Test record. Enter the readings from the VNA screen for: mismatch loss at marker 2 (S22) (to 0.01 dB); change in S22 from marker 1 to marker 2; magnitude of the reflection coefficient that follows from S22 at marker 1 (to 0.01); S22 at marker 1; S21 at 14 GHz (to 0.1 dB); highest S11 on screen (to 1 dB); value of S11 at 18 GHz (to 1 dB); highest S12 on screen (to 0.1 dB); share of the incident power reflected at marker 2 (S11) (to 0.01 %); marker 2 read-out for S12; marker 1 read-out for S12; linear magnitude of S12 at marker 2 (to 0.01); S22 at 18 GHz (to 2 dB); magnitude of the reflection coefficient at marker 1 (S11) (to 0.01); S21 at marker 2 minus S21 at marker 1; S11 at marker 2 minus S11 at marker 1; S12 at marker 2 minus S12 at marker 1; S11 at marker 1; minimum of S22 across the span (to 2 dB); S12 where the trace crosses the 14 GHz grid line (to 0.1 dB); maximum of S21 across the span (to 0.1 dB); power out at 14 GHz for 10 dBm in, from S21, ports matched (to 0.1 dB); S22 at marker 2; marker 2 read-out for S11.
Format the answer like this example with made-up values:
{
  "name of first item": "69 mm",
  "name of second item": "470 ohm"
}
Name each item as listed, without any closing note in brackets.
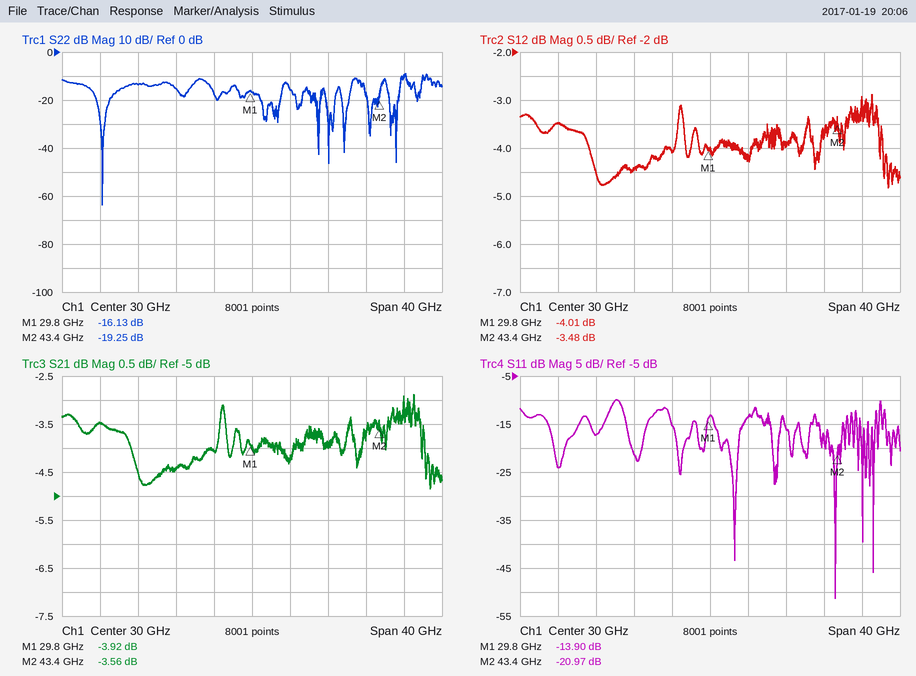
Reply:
{
  "mismatch loss at marker 2 (S22)": "0.05 dB",
  "change in S22 from marker 1 to marker 2": "-3.12 dB",
  "magnitude of the reflection coefficient that follows from S22 at marker 1": "0.16",
  "S22 at marker 1": "-16.13 dB",
  "S21 at 14 GHz": "-3.5 dB",
  "highest S11 on screen": "-10 dB",
  "value of S11 at 18 GHz": "-17 dB",
  "highest S12 on screen": "-2.9 dB",
  "share of the incident power reflected at marker 2 (S11)": "0.80 %",
  "marker 2 read-out for S12": "-3.48 dB",
  "marker 1 read-out for S12": "-4.01 dB",
  "linear magnitude of S12 at marker 2": "0.67",
  "S22 at 18 GHz": "-14 dB",
  "magnitude of the reflection coefficient at marker 1 (S11)": "0.20",
  "S21 at marker 2 minus S21 at marker 1": "0.36 dB",
  "S11 at marker 2 minus S11 at marker 1": "-7.07 dB",
  "S12 at marker 2 minus S12 at marker 1": "0.53 dB",
  "S11 at marker 1": "-13.90 dB",
  "minimum of S22 across the span": "-64 dB",
  "S12 where the trace crosses the 14 GHz grid line": "-3.5 dB",
  "maximum of S21 across the span": "-2.9 dB",
  "power out at 14 GHz for 10 dBm in, from S21, ports matched": "6.5 dBm",
  "S22 at marker 2": "-19.25 dB",
  "marker 2 read-out for S11": "-20.97 dB"
}
